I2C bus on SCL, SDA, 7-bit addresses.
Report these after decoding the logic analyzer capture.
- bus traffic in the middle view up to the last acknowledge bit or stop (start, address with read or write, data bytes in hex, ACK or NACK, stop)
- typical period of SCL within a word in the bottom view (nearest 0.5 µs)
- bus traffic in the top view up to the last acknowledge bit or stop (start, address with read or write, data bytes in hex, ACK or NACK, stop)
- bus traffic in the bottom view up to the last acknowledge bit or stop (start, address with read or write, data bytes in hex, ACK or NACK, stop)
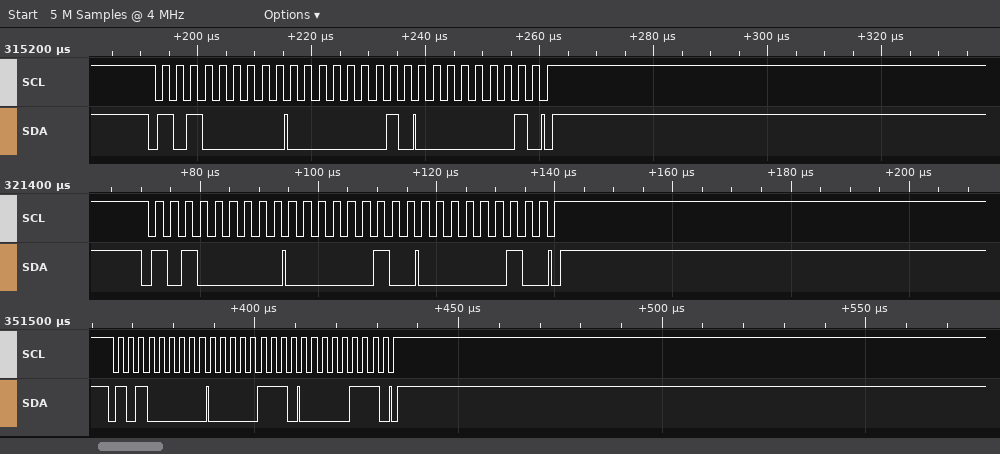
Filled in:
start, address 50 write ACK, 02 ACK, 02 ACK, stop
2.5 µs
start, address 50 write ACK, 01 ACK, 01 ACK, stop
start, address 50 write ACK, 07 ACK, 07 ACK, stop
